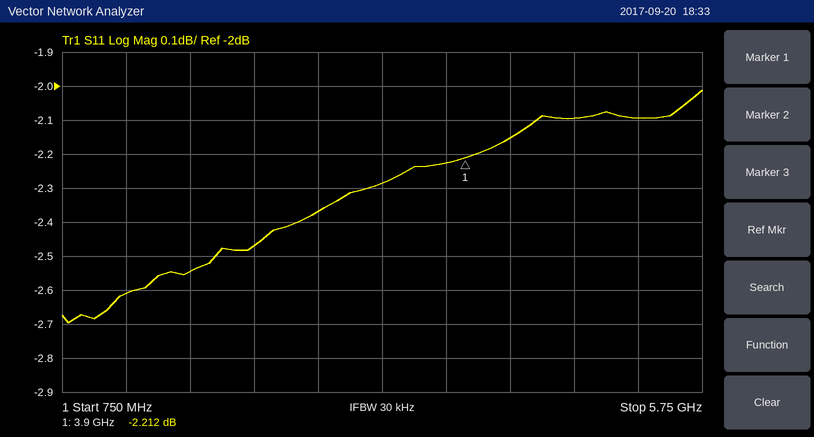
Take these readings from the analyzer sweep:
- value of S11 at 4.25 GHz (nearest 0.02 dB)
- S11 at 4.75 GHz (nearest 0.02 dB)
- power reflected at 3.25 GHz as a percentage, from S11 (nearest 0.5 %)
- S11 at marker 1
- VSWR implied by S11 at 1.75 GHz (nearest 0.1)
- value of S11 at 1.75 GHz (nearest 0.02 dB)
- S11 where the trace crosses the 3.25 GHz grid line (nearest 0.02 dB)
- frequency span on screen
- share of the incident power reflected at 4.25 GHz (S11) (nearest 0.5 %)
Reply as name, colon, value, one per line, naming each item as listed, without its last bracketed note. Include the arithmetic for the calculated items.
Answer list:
value of S11 at 4.25 GHz: -2.16 dB
S11 at 4.75 GHz: -2.10 dB
power reflected at 3.25 GHz as a percentage, from S11: 10^(-2.28/10) ≈ 59.2 %, so 59.0 % to the nearest 0.5 %
S11 at marker 1: -2.212 dB
VSWR implied by S11 at 1.75 GHz: |Γ| = 10^(-2.54/20) = 0.7464; VSWR = (1 + 0.7464)/(1 − 0.7464) ≈ 6.9
value of S11 at 1.75 GHz: -2.54 dB
S11 where the trace crosses the 3.25 GHz grid line: -2.28 dB
frequency span on screen: 5 GHz
share of the incident power reflected at 4.25 GHz (S11): 10^(-2.16/10) ≈ 60.8 %, so 61.0 % to the nearest 0.5 %
